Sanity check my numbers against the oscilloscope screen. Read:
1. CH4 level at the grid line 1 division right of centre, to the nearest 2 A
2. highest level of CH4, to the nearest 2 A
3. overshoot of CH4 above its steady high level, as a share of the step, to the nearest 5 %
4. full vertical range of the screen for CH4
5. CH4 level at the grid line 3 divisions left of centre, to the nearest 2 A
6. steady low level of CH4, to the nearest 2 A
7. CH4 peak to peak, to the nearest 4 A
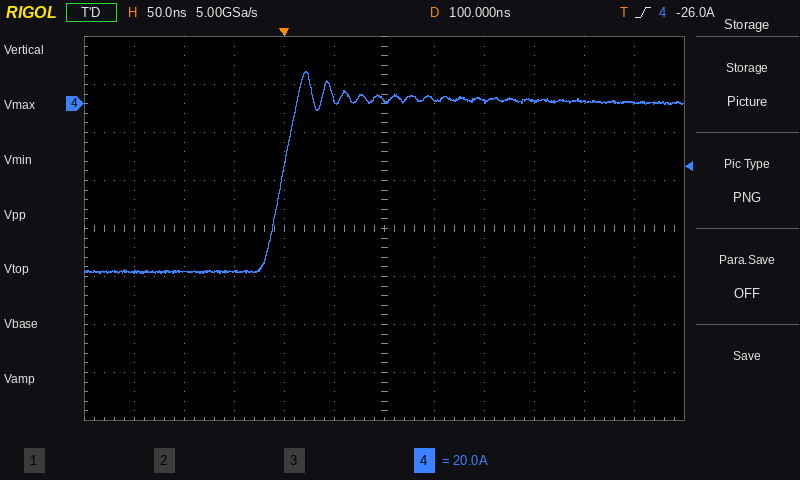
2 A
14 A
20 %
160 A
-70 A
-70 A
84 A
